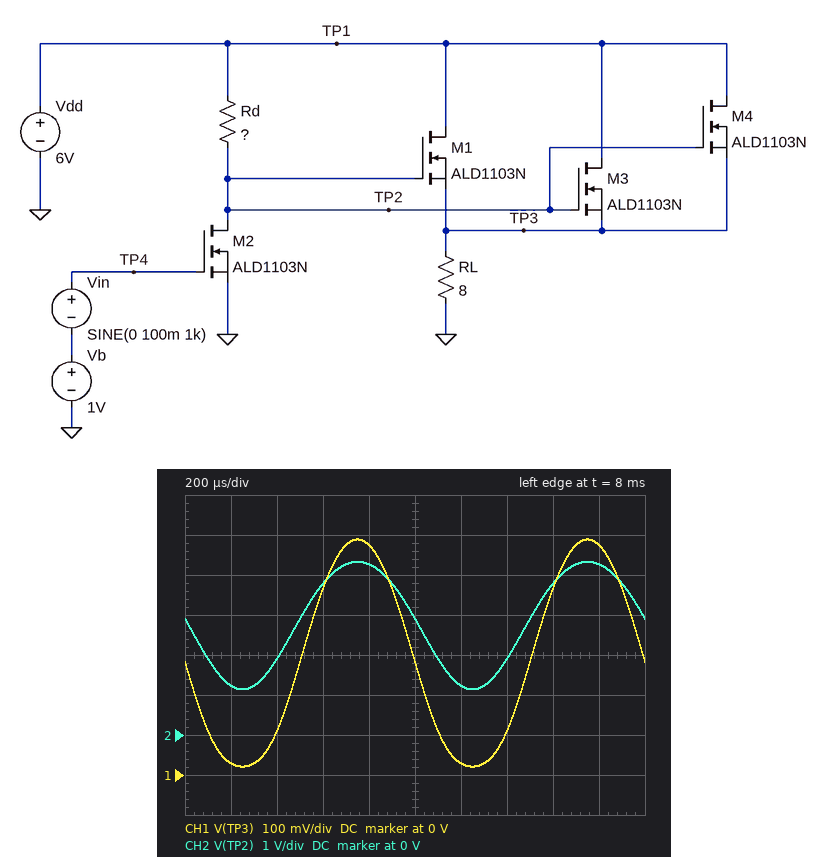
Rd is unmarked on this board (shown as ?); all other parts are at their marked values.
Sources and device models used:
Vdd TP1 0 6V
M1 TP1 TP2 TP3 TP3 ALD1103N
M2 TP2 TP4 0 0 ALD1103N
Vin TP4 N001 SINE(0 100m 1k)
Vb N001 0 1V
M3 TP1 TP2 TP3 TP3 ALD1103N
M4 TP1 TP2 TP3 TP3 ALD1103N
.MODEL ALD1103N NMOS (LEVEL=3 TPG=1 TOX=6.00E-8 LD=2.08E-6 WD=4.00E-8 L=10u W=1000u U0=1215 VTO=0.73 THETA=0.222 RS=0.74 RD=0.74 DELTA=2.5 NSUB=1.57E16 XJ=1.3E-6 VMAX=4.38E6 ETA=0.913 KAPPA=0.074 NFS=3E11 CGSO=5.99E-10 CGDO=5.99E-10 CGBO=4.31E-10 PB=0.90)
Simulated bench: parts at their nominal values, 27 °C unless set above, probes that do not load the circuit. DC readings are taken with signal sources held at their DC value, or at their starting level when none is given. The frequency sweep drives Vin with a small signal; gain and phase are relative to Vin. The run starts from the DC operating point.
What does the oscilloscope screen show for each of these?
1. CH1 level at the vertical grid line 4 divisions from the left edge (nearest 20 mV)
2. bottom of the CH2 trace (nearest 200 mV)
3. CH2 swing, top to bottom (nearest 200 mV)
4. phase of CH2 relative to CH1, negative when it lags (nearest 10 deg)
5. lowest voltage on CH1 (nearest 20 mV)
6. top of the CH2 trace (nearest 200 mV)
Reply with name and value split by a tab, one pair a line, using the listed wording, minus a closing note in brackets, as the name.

CH1 level at the vertical grid line 4 divisions from the left edge	580 mV
bottom of the CH2 trace	1.2 V
CH2 swing, top to bottom	3.2 V
phase of CH2 relative to CH1, negative when it lags	0 deg
lowest voltage on CH1	20 mV
top of the CH2 trace	4.4 V
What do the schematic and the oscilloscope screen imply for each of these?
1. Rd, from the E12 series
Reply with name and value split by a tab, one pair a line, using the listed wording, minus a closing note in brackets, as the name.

Rd, from the E12 series	6.8 kΩ
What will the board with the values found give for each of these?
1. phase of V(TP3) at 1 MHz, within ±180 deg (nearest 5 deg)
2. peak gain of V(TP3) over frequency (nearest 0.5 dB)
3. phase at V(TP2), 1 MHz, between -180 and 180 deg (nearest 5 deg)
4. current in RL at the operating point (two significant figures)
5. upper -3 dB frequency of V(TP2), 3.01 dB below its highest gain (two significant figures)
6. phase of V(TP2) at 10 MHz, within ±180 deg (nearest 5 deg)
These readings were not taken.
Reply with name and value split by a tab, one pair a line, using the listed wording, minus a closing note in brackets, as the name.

phase of V(TP3) at 1 MHz, within ±180 deg	160 deg
peak gain of V(TP3) over frequency	10.0 dB
phase at V(TP2), 1 MHz, between -180 and 180 deg	160 deg
current in RL at the operating point	35 mA
upper -3 dB frequency of V(TP2), 3.01 dB below its highest gain	2.8 MHz
phase of V(TP2) at 10 MHz, within ±180 deg	105 deg
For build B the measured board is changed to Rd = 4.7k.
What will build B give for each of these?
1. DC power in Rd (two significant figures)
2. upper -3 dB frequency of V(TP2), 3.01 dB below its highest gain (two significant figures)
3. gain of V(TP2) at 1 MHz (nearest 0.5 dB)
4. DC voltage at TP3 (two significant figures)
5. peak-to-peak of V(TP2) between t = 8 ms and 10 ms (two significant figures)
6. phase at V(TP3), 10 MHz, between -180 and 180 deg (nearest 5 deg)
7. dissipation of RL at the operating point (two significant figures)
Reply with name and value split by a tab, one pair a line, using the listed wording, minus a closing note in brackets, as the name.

DC power in Rd	1.0 mW
upper -3 dB frequency of V(TP2), 3.01 dB below its highest gain	4.1 MHz
gain of V(TP2) at 1 MHz	21.0 dB
DC voltage at TP3	470 mV
peak-to-peak of V(TP2) between t = 8 ms and 10 ms	2.3 V
phase at V(TP3), 10 MHz, between -180 and 180 deg	110 deg
dissipation of RL at the operating point	27 mW
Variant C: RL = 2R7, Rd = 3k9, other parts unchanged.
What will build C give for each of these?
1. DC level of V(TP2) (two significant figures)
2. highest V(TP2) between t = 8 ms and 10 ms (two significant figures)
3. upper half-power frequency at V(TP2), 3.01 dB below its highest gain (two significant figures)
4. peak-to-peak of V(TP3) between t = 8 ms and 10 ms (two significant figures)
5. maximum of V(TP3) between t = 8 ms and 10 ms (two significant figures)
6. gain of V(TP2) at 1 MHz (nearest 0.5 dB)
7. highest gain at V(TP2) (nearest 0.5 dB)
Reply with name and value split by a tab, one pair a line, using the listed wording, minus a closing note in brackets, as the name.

DC level of V(TP2)	4.1 V
highest V(TP2) between t = 8 ms and 10 ms	5.0 V
upper half-power frequency at V(TP2), 3.01 dB below its highest gain	4.3 MHz
peak-to-peak of V(TP3) between t = 8 ms and 10 ms	180 mV
maximum of V(TP3) between t = 8 ms and 10 ms	300 mV
gain of V(TP2) at 1 MHz	19.5 dB
highest gain at V(TP2)	20.0 dB
